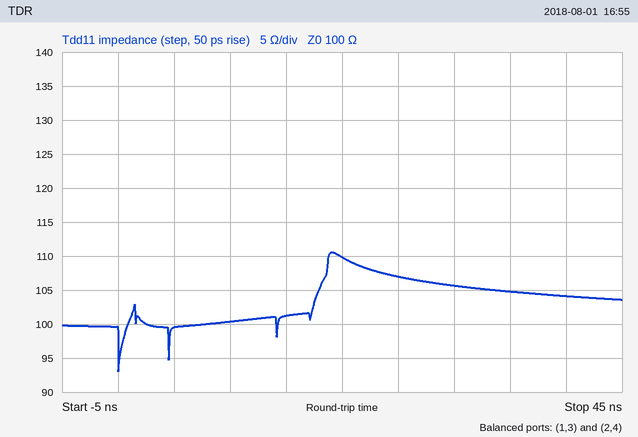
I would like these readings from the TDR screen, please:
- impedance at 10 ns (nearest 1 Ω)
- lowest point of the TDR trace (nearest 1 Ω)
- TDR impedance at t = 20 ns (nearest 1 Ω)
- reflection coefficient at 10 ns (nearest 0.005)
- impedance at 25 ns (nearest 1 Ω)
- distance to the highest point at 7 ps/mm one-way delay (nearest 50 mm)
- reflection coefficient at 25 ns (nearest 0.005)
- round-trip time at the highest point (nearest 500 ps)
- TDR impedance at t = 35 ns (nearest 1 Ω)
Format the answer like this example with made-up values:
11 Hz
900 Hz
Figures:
100 Ω
93 Ω
110 Ω
0.000
107 Ω
1.35 m
+0.035
19.0 ns
105 Ω
